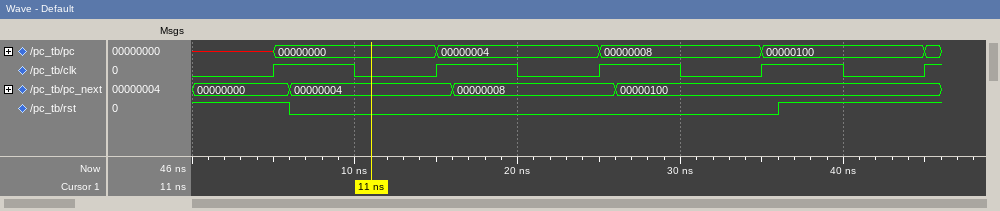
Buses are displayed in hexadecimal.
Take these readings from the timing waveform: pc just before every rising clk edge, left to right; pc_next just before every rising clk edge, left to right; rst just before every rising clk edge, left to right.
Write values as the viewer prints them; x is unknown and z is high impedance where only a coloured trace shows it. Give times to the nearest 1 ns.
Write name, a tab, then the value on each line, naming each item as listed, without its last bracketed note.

pc just before every rising clk edge, left to right	x, 00000000, 00000004, 00000008, 00000100
pc_next just before every rising clk edge, left to right	00000000, 00000004, 00000008, 00000100, 00000100
rst just before every rising clk edge, left to right	1 0 0 0 1
